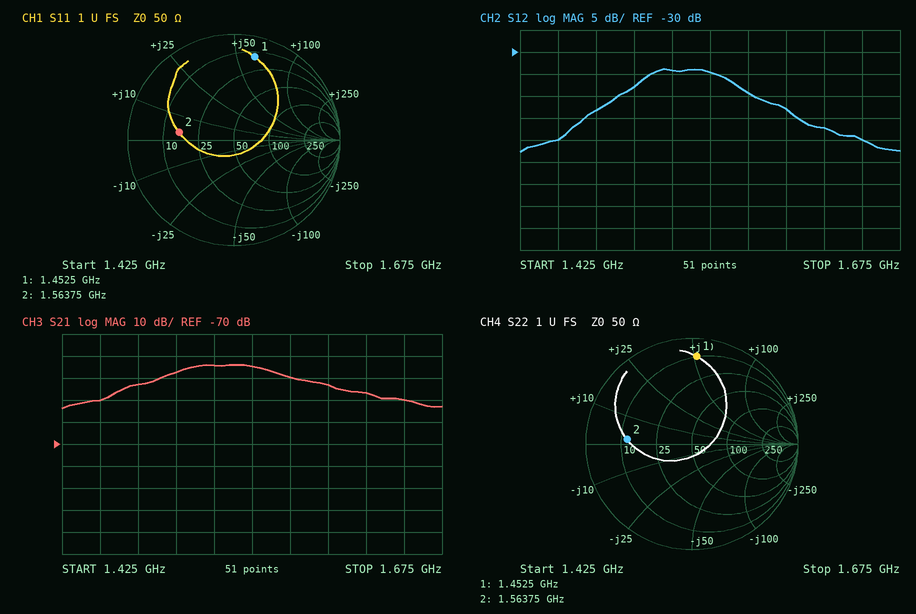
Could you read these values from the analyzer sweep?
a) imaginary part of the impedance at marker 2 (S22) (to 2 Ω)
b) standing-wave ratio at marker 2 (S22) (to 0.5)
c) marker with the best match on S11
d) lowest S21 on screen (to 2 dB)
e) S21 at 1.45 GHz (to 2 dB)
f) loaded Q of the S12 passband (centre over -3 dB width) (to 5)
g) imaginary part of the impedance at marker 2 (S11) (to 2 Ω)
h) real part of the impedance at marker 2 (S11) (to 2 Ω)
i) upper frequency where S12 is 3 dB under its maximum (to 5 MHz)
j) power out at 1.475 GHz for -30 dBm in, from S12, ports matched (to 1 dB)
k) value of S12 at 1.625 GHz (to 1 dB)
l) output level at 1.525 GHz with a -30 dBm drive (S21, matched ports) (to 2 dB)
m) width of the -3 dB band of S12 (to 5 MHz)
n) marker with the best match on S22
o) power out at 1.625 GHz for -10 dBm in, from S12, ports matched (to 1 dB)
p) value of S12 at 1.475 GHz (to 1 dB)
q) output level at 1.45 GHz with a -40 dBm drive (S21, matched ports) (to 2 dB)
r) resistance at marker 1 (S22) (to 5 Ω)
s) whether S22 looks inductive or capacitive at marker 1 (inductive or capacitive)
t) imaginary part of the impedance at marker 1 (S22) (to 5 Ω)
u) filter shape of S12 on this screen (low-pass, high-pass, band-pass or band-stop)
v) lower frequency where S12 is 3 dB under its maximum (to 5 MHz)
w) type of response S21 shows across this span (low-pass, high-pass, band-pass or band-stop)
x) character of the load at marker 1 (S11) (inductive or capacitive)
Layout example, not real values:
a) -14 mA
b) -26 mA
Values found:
a) +2 Ω
b) 4.0
c) marker 2
d) -54 dB
e) -50 dB
f) 25
g) +4 Ω
h) 16 Ω
i) 1.565 GHz
j) -73 dBm
k) -47 dB
l) -64 dBm
m) 60 MHz
n) marker 2
o) -57 dBm
p) -43 dB
q) -90 dBm
r) 10 Ω
s) inductive
t) +50 Ω
u) band-pass
v) 1.505 GHz
w) band-pass
x) inductive
